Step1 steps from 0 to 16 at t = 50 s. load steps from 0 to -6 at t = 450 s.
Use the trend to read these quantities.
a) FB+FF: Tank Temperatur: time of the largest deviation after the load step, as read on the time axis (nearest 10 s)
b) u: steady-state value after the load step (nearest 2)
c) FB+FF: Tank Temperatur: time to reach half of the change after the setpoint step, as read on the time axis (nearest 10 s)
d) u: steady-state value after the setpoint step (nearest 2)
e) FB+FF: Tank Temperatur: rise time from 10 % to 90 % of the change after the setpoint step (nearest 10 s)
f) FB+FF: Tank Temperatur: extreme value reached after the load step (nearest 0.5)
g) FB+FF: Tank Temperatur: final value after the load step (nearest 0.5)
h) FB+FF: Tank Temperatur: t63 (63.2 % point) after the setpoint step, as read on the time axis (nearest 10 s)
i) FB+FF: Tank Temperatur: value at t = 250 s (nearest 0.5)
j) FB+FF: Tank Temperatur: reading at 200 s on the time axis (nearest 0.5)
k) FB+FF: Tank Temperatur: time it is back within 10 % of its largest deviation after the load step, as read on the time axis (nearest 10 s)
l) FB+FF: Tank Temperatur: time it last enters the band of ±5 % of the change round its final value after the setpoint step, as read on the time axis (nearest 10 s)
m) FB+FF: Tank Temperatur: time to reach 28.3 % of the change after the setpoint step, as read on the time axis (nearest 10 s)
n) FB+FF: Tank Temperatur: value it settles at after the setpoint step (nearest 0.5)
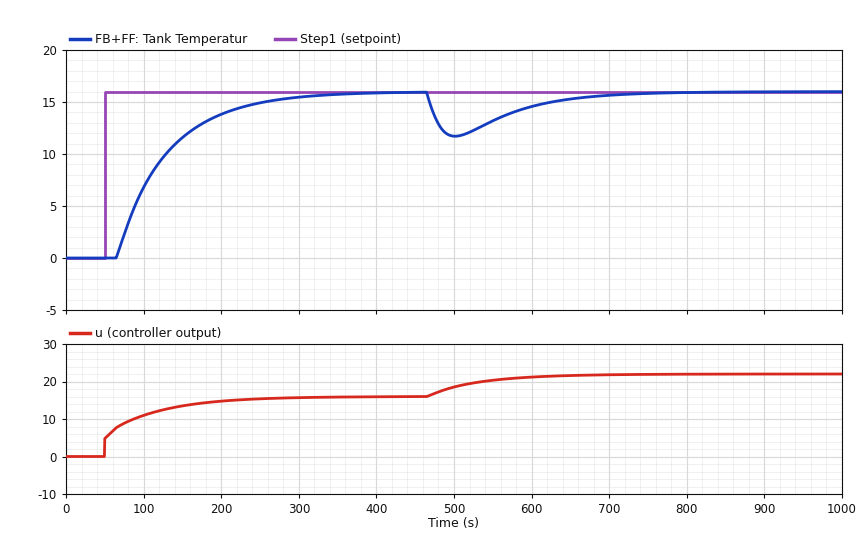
500 s
22
110 s
16
150 s
11.5
16.0
130 s
15.0
14.0
690 s
270 s
90 s
16.0
